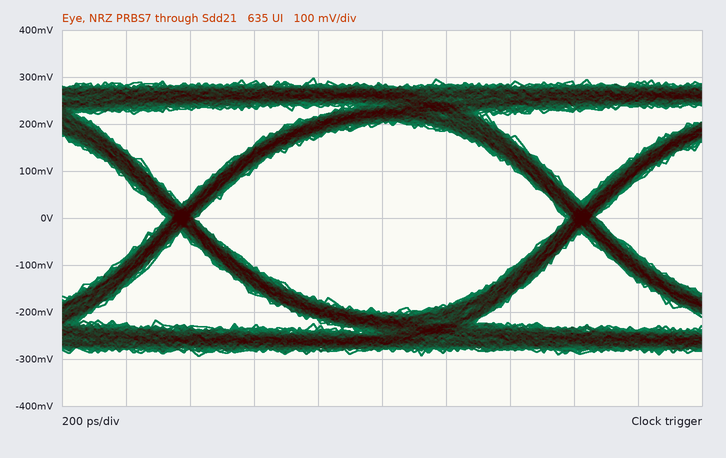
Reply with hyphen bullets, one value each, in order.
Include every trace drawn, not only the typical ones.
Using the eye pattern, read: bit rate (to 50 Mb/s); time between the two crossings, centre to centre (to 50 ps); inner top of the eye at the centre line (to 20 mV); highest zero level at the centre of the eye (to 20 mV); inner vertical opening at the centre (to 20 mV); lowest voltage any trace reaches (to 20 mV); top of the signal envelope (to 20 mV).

- 800 Mb/s
- 1.25 ns
- 200 mV
- -200 mV
- 400 mV
- -300 mV
- 300 mV
